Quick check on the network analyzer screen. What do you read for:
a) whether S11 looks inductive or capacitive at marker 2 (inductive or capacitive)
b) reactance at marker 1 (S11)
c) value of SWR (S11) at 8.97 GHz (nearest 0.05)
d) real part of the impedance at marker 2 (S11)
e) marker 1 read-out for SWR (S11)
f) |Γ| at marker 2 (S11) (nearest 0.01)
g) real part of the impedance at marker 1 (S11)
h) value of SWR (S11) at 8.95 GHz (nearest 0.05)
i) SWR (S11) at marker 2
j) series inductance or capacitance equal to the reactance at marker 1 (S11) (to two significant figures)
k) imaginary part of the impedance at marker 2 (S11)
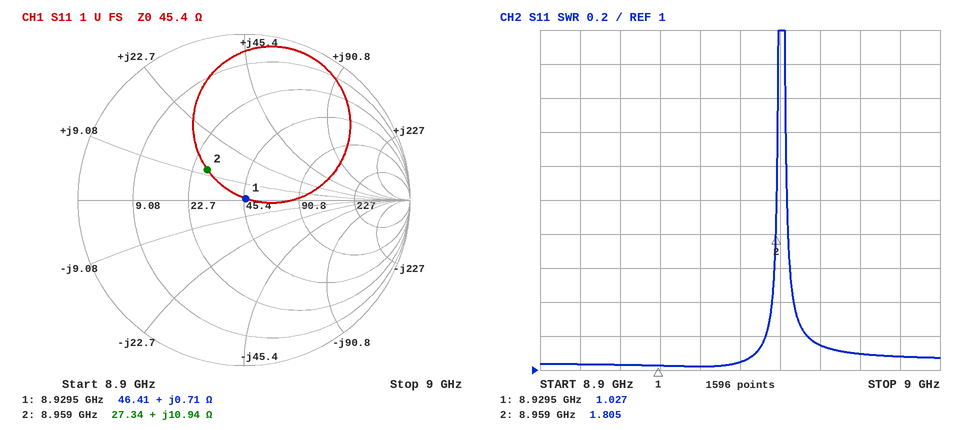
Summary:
inductive
+0.71 Ω
1.15
27.34 Ω
1.027
0.29
46.41 Ω
1.05
1.805
13 pH
+10.94 Ω
